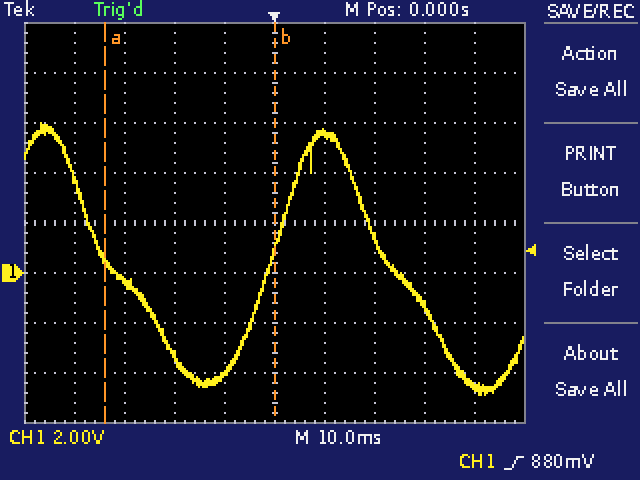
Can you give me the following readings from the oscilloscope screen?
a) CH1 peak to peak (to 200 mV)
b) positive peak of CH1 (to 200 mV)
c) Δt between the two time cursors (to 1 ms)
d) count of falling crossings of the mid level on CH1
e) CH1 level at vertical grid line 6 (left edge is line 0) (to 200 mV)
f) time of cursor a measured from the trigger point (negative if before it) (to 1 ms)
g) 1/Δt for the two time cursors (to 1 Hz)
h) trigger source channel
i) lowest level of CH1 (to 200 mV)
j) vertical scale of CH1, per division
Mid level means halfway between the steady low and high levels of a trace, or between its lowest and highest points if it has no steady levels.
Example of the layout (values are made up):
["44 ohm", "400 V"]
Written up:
["10.8 V", "6.0 V", "34 ms", "2", "5.6 V", "-34 ms", "29 Hz", "CH1", "-4.8 V", "2 V"]
